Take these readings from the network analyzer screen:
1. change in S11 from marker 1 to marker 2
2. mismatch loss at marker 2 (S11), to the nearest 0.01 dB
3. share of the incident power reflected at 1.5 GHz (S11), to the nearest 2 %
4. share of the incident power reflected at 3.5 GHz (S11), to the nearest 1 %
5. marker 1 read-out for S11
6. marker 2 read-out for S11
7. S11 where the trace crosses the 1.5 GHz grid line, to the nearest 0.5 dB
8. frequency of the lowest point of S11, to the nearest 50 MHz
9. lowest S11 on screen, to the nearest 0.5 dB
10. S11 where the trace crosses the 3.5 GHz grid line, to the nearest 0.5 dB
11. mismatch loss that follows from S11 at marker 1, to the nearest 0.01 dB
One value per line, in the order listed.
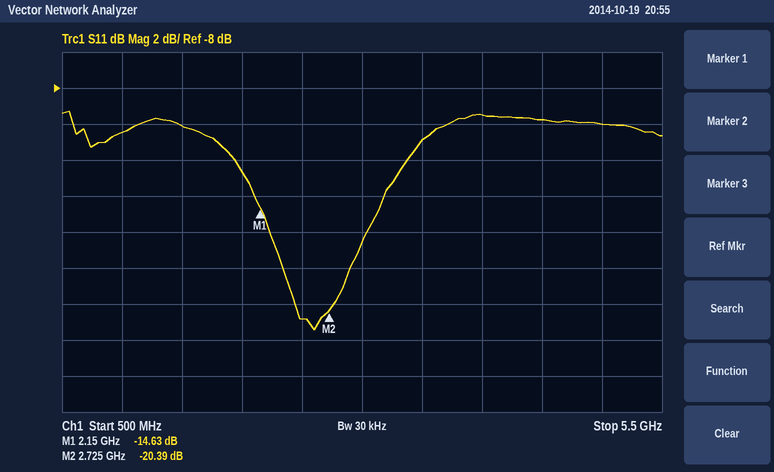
-5.76 dB
0.04 dB
10 %
8 %
-14.63 dB
-20.39 dB
-10.0 dB
2.60 GHz
-21.5 dB
-11.0 dB
0.15 dB
